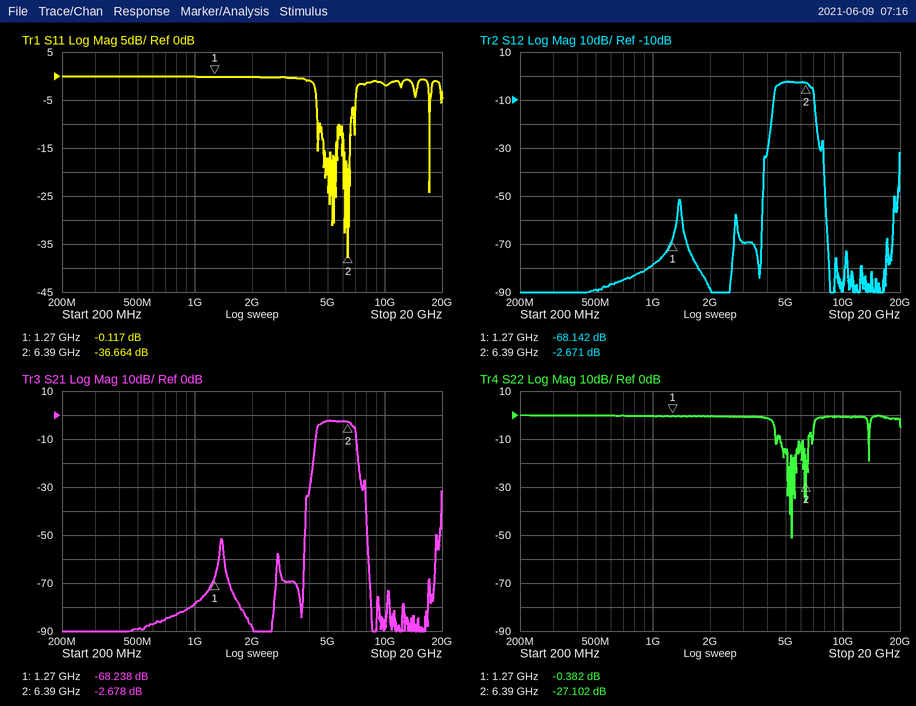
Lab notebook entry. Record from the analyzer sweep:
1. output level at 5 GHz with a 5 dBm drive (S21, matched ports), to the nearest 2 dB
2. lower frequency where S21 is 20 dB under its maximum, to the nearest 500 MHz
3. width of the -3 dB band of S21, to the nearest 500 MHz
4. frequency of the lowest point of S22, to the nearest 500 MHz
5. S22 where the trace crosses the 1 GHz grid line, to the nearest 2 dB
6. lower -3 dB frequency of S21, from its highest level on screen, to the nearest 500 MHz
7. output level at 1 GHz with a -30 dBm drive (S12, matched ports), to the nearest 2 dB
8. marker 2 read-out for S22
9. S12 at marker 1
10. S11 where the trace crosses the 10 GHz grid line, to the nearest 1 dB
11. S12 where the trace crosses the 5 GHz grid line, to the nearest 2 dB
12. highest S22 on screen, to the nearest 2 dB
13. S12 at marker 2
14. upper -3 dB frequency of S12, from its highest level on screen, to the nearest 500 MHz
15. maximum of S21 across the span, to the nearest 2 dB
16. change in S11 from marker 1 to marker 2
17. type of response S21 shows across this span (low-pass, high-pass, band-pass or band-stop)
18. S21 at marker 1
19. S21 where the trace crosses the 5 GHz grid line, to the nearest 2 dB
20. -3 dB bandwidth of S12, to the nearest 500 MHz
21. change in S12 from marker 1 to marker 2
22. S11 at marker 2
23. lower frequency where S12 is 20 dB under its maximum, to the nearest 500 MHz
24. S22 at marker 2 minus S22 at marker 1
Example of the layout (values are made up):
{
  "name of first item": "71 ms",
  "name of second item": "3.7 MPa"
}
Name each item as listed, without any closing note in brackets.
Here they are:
{
  "output level at 5 GHz with a 5 dBm drive (S21, matched ports), to the nearest 2 dB": "2 dBm",
  "lower frequency where S21 is 20 dB under its maximum, to the nearest 500 MHz": "4.0 GHz",
  "width of the -3 dB band of S21, to the nearest 500 MHz": "2.5 GHz",
  "frequency of the lowest point of S22, to the nearest 500 MHz": "5.5 GHz",
  "S22 where the trace crosses the 1 GHz grid line, to the nearest 2 dB": "0 dB",
  "lower -3 dB frequency of S21, from its highest level on screen, to the nearest 500 MHz": "4.5 GHz",
  "output level at 1 GHz with a -30 dBm drive (S12, matched ports), to the nearest 2 dB": "-108 dBm",
  "marker 2 read-out for S22": "-27.102 dB",
  "S12 at marker 1": "-68.142 dB",
  "S11 where the trace crosses the 10 GHz grid line, to the nearest 1 dB": "-2 dB",
  "S12 where the trace crosses the 5 GHz grid line, to the nearest 2 dB": "-2 dB",
  "highest S22 on screen, to the nearest 2 dB": "0 dB",
  "S12 at marker 2": "-2.671 dB",
  "upper -3 dB frequency of S12, from its highest level on screen, to the nearest 500 MHz": "7.0 GHz",
  "maximum of S21 across the span, to the nearest 2 dB": "-2 dB",
  "change in S11 from marker 1 to marker 2": "-36.547 dB",
  "type of response S21 shows across this span": "band-pass",
  "S21 at marker 1": "-68.238 dB",
  "S21 where the trace crosses the 5 GHz grid line, to the nearest 2 dB": "-2 dB",
  "-3 dB bandwidth of S12, to the nearest 500 MHz": "2.5 GHz",
  "change in S12 from marker 1 to marker 2": "65.471 dB",
  "S11 at marker 2": "-36.664 dB",
  "lower frequency where S12 is 20 dB under its maximum, to the nearest 500 MHz": "4.0 GHz",
  "S22 at marker 2 minus S22 at marker 1": "-26.720 dB"
}
